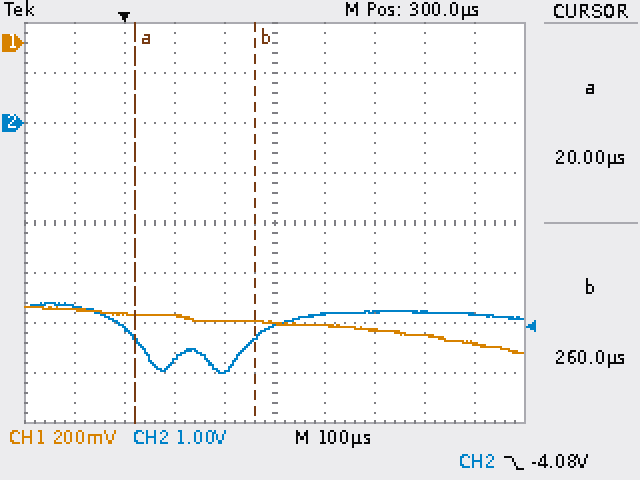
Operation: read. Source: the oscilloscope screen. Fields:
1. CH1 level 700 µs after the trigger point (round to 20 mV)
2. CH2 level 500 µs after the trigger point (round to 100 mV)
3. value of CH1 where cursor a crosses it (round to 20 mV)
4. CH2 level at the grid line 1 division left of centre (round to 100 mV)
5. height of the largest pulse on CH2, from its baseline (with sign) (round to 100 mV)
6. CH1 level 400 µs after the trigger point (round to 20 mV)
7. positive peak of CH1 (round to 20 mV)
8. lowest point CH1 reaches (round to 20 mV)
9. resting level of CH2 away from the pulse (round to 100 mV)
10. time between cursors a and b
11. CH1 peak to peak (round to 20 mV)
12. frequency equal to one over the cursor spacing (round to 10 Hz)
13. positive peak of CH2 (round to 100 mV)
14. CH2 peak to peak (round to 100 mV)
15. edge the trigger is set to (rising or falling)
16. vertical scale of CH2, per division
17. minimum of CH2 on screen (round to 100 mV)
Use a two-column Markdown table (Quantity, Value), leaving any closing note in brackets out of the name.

| Quantity | Value |
|---|---|
| CH1 level 700 µs after the trigger point | -1.20 V |
| CH2 level 500 µs after the trigger point | -3.8 V |
| value of CH1 where cursor a crosses it | -1.08 V |
| CH2 level at the grid line 1 division left of centre | -5.0 V |
| height of the largest pulse on CH2, from its baseline (with sign) | -1.2 V |
| CH1 level 400 µs after the trigger point | -1.12 V |
| positive peak of CH1 | -1.06 V |
| lowest point CH1 reaches | -1.24 V |
| resting level of CH2 away from the pulse | -3.8 V |
| time between cursors a and b | 240 µs |
| CH1 peak to peak | 180 mV |
| frequency equal to one over the cursor spacing | 4.17 kHz |
| positive peak of CH2 | -3.6 V |
| CH2 peak to peak | 1.4 V |
| edge the trigger is set to | falling |
| vertical scale of CH2, per division | 1 V |
| minimum of CH2 on screen | -5.0 V |
